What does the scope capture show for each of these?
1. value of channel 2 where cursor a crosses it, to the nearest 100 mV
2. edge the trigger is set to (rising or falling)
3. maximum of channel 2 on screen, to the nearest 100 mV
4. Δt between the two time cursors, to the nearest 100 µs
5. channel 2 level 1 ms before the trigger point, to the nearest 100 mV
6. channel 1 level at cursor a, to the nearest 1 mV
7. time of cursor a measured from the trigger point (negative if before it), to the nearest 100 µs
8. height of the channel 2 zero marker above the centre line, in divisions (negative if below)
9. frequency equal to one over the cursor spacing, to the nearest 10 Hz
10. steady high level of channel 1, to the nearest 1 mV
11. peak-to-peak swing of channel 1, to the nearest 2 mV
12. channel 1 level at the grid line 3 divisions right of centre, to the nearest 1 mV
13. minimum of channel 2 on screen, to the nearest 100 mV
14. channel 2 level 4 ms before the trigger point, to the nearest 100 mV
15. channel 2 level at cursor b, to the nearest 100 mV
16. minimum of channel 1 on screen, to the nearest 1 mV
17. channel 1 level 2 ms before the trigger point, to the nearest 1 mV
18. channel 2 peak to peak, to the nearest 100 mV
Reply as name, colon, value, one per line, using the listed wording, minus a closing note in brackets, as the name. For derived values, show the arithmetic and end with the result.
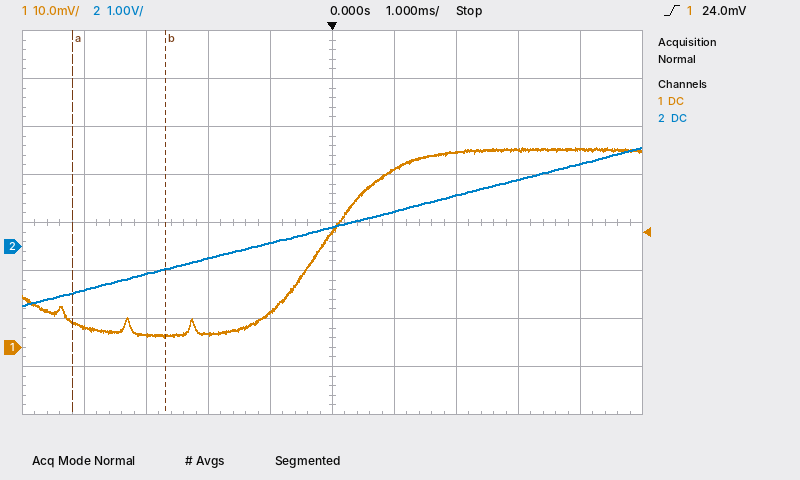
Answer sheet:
value of channel 2 where cursor a crosses it, to the nearest 100 mV: -1.0 V
edge the trigger is set to: rising
maximum of channel 2 on screen, to the nearest 100 mV: 2.1 V
Δt between the two time cursors, to the nearest 100 µs: 1.5 ms
channel 2 level 1 ms before the trigger point, to the nearest 100 mV: 100 mV
channel 1 level at cursor a, to the nearest 1 mV: 5 mV
time of cursor a measured from the trigger point (negative if before it), to the nearest 100 µs: -4.2 ms
height of the channel 2 zero marker above the centre line, in divisions: -0.5 div
frequency equal to one over the cursor spacing, to the nearest 10 Hz: 1 / 1.5 ms ≈ 670 Hz
steady high level of channel 1, to the nearest 1 mV: 41 mV
peak-to-peak swing of channel 1, to the nearest 2 mV: 40 mV
channel 1 level at the grid line 3 divisions right of centre, to the nearest 1 mV: 41 mV
minimum of channel 2 on screen, to the nearest 100 mV: -1.2 V
channel 2 level 4 ms before the trigger point, to the nearest 100 mV: -900 mV
channel 2 level at cursor b, to the nearest 100 mV: -500 mV
minimum of channel 1 on screen, to the nearest 1 mV: 2 mV
channel 1 level 2 ms before the trigger point, to the nearest 1 mV: 3 mV
channel 2 peak to peak, to the nearest 100 mV: 2.1 V − (-1.2 V) = 3.3 V
